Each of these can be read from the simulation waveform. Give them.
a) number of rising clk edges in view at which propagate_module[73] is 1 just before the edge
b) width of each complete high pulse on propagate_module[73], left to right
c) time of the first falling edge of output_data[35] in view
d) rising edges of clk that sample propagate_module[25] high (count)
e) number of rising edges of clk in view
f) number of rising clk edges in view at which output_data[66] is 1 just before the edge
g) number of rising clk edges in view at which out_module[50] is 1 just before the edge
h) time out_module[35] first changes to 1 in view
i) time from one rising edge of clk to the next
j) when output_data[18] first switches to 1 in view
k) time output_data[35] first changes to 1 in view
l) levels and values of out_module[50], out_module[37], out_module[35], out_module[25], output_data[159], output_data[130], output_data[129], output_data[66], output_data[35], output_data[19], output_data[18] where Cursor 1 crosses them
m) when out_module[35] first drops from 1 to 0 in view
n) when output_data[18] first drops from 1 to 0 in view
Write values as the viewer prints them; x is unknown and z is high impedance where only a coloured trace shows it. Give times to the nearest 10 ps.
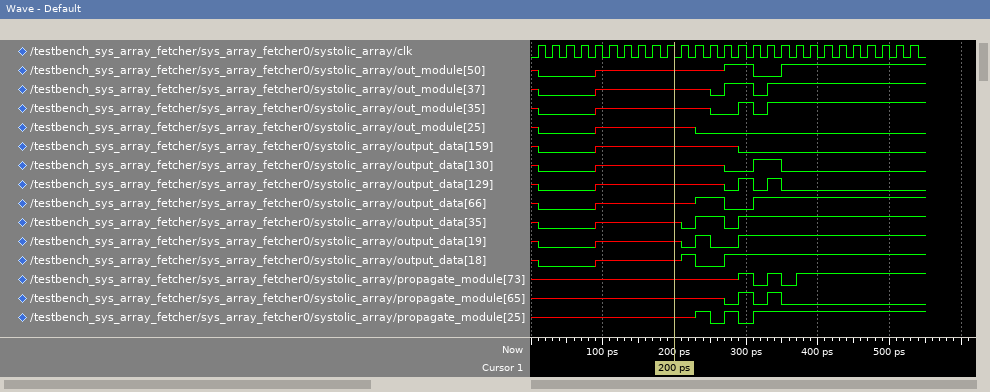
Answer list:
10
20 ps
270 ps
13
27
13
11
290 ps
20 ps
210 ps
230 ps
out_module[50]=x, out_module[37]=x, out_module[35]=x, out_module[25]=x, output_data[159]=x, output_data[130]=x, output_data[129]=x, output_data[66]=x, output_data[35]=x, output_data[19]=x, output_data[18]=x
310 ps
230 ps
